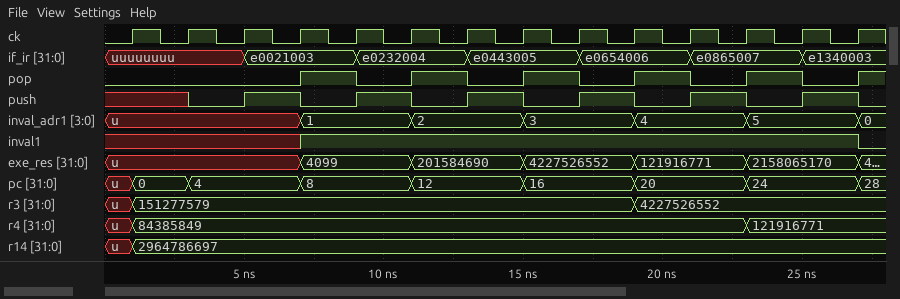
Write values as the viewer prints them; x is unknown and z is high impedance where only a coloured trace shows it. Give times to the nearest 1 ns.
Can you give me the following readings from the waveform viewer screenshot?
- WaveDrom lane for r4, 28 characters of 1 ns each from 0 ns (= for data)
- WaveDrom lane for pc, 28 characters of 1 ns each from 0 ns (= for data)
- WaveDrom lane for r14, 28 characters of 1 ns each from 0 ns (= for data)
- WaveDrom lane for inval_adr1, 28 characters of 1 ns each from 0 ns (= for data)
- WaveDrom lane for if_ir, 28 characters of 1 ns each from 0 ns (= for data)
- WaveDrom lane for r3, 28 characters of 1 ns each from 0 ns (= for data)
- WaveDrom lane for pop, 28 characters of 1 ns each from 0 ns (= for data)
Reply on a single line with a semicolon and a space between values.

{name: 'r4', wave: 'x=.....................=....', data: '84385849 121916771'}; {name: 'pc', wave: 'x=.=...=...=...=...=...=...=', data: '0 4 8 12 16 20 24 28'}; {name: 'r14', wave: 'x=..........................', data: '2964786697'}; {name: 'inval_adr1', wave: 'x......=...=...=...=...=...=', data: '1 2 3 4 5 0'}; {name: 'if_ir', wave: 'x....=...=...=...=...=...=..', data: 'e0021003 e0232004 e0443005 e0654006 e0865007 e1340003'}; {name: 'r3', wave: 'x=.................=........', data: '151277579 4227526552'}; {name: 'pop', wave: '0......1.0.1.0.1.0.1.0.1.0.1'}
